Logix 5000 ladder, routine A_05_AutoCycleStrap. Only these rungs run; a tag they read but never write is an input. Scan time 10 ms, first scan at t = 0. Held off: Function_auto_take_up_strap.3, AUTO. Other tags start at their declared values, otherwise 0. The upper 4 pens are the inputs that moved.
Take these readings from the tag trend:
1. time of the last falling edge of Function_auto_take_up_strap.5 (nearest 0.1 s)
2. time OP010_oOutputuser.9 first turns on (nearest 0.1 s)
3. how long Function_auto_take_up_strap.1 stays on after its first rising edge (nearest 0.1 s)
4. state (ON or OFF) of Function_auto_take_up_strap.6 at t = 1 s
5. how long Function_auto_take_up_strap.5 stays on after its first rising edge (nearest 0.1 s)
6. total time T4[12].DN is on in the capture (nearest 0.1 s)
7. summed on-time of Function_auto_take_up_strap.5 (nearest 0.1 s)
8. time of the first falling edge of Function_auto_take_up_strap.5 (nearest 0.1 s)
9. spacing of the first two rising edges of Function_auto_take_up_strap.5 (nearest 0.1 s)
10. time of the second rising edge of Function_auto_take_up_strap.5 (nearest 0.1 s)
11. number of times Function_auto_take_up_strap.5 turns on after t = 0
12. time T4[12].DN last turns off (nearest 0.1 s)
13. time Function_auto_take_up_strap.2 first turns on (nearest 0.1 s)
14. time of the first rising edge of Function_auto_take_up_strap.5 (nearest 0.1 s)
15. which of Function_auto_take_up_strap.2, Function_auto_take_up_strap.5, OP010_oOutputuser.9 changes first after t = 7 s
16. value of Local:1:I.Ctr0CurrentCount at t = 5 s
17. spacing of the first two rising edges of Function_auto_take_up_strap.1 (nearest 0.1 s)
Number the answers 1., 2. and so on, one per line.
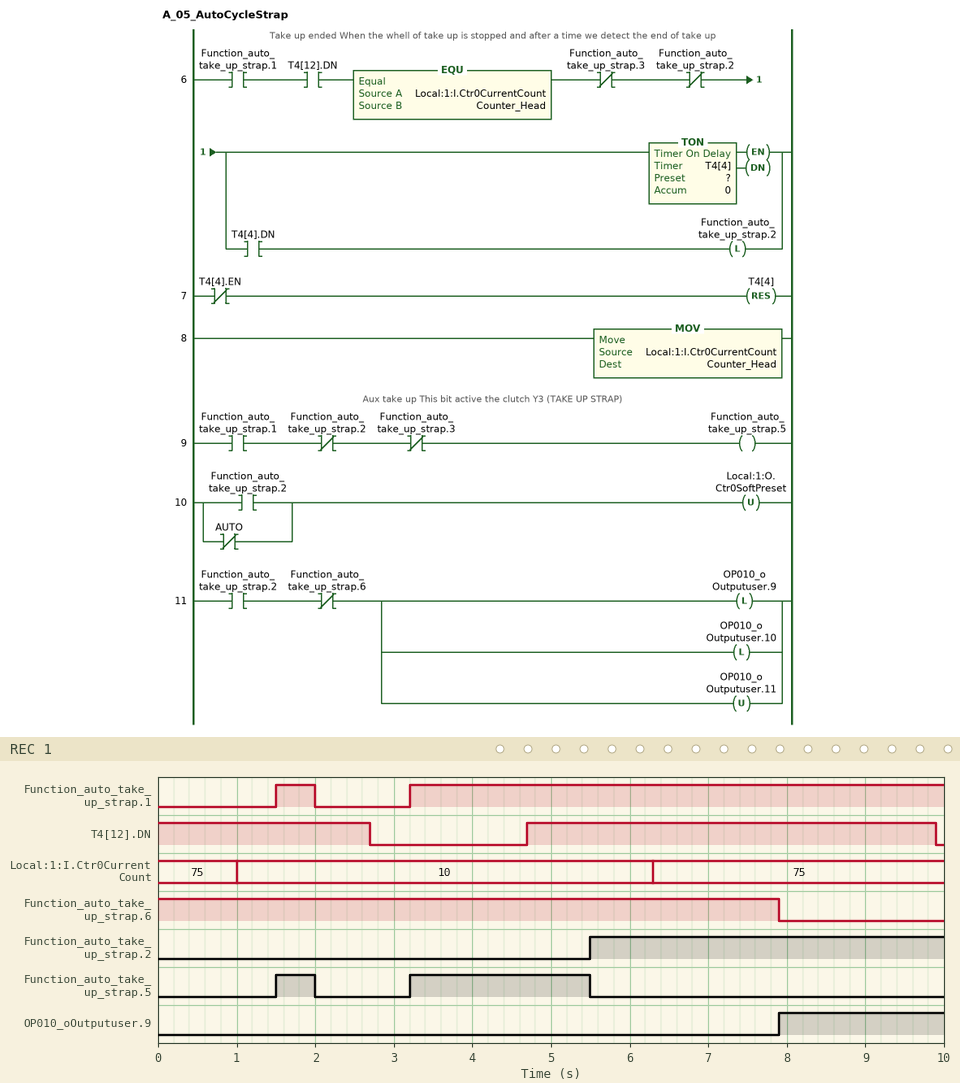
1. 5.5 s
2. 7.9 s
3. 0.5 s
4. ON
5. 0.5 s
6. 7.9 s
7. 2.8 s
8. 2.0 s
9. 1.7 s
10. 3.2 s
11. 2
12. 9.9 s
13. 5.5 s
14. 1.5 s
15. OP010_oOutputuser.9
16. 10
17. 1.7 s
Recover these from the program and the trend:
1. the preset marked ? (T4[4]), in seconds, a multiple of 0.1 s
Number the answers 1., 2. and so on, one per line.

1. 0.8 s
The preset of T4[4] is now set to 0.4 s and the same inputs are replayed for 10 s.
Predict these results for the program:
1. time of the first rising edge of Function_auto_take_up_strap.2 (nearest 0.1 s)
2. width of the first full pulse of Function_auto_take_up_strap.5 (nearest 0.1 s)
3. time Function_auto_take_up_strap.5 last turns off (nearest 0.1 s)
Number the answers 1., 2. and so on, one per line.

1. 1.9 s
2. 0.4 s
3. 1.9 s
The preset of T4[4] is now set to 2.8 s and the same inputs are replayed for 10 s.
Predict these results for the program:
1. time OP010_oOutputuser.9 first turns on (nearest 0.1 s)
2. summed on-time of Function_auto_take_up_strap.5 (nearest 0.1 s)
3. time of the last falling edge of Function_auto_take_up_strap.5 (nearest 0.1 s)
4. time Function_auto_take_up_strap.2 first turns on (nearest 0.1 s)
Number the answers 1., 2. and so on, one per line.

1. 9.1 s
2. 6.4 s
3. 9.1 s
4. 9.1 s
